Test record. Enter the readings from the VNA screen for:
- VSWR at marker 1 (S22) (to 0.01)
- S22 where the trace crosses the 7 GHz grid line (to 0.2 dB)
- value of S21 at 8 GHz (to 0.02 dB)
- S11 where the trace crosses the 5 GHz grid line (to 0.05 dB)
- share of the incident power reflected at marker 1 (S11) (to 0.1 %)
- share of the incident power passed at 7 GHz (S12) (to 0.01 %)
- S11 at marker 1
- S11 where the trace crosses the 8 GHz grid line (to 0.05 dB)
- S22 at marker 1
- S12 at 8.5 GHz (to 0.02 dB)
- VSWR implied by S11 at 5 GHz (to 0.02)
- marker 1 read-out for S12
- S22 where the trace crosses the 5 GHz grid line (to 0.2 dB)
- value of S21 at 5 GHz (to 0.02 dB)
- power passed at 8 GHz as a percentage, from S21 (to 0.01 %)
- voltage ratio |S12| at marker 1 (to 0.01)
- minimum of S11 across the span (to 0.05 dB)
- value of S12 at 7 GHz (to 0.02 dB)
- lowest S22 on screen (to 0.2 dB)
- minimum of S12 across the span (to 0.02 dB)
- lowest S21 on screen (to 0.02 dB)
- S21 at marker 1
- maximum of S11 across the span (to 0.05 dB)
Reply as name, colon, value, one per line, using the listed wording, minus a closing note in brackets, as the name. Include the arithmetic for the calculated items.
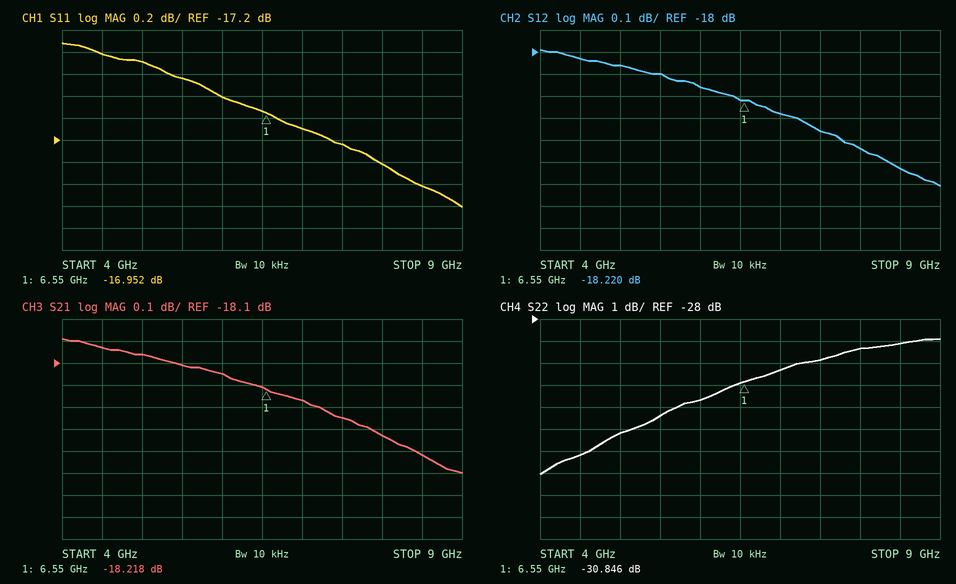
VSWR at marker 1 (S22): (1 + 0.0287)/(1 − 0.0287) ≈ 1.06
S22 where the trace crosses the 7 GHz grid line: -30.4 dB
value of S21 at 8 GHz: -18.42 dB
S11 where the trace crosses the 5 GHz grid line: -16.50 dB
share of the incident power reflected at marker 1 (S11): 10^(-16.952/10) ≈ 2.0 %
share of the incident power passed at 7 GHz (S12): 10^(-18.28/10) ≈ 1.49 %
S11 at marker 1: -16.952 dB
S11 where the trace crosses the 8 GHz grid line: -17.40 dB
S22 at marker 1: -30.846 dB
S12 at 8.5 GHz: -18.52 dB
VSWR implied by S11 at 5 GHz: |Γ| = 10^(-16.5/20) = 0.1496; VSWR = (1 + 0.1496)/(1 − 0.1496) ≈ 1.35, so 1.36 to the nearest 0.02
marker 1 read-out for S12: -18.220 dB
S22 where the trace crosses the 5 GHz grid line: -33.2 dB
value of S21 at 5 GHz: -18.06 dB
power passed at 8 GHz as a percentage, from S21: 10^(-18.42/10) ≈ 1.44 %
voltage ratio |S12| at marker 1: 10^(-18.22/20) ≈ 0.12
minimum of S11 across the span: -17.80 dB
value of S12 at 7 GHz: -18.28 dB
lowest S22 on screen: -35.0 dB
minimum of S12 across the span: -18.60 dB
lowest S21 on screen: -18.60 dB
S21 at marker 1: -18.218 dB
maximum of S11 across the span: -16.30 dB
